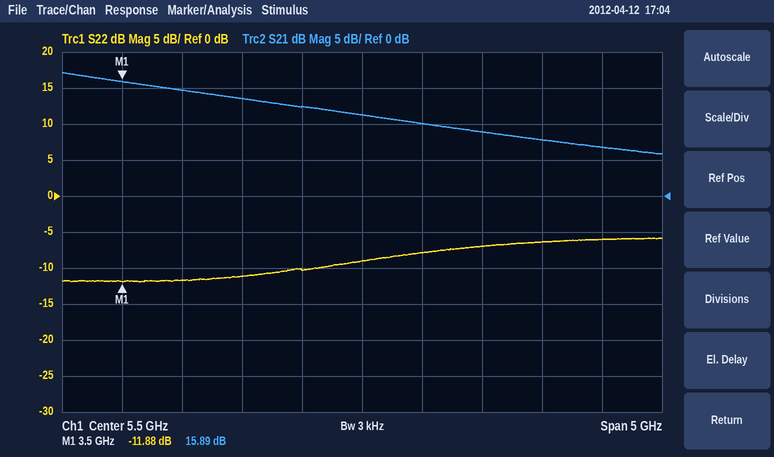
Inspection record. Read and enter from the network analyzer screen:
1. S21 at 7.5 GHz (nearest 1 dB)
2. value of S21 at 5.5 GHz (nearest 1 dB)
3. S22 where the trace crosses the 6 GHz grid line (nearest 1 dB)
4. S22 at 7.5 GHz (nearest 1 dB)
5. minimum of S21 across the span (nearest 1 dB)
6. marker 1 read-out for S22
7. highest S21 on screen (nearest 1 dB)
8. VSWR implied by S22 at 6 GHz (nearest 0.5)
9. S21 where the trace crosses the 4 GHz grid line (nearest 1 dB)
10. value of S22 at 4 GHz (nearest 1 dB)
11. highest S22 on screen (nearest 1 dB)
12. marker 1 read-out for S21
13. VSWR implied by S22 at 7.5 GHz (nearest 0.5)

7 dB
11 dB
-8 dB
-6 dB
6 dB
-11.88 dB
17 dB
2.5
15 dB
-12 dB
-6 dB
15.89 dB
3.0
